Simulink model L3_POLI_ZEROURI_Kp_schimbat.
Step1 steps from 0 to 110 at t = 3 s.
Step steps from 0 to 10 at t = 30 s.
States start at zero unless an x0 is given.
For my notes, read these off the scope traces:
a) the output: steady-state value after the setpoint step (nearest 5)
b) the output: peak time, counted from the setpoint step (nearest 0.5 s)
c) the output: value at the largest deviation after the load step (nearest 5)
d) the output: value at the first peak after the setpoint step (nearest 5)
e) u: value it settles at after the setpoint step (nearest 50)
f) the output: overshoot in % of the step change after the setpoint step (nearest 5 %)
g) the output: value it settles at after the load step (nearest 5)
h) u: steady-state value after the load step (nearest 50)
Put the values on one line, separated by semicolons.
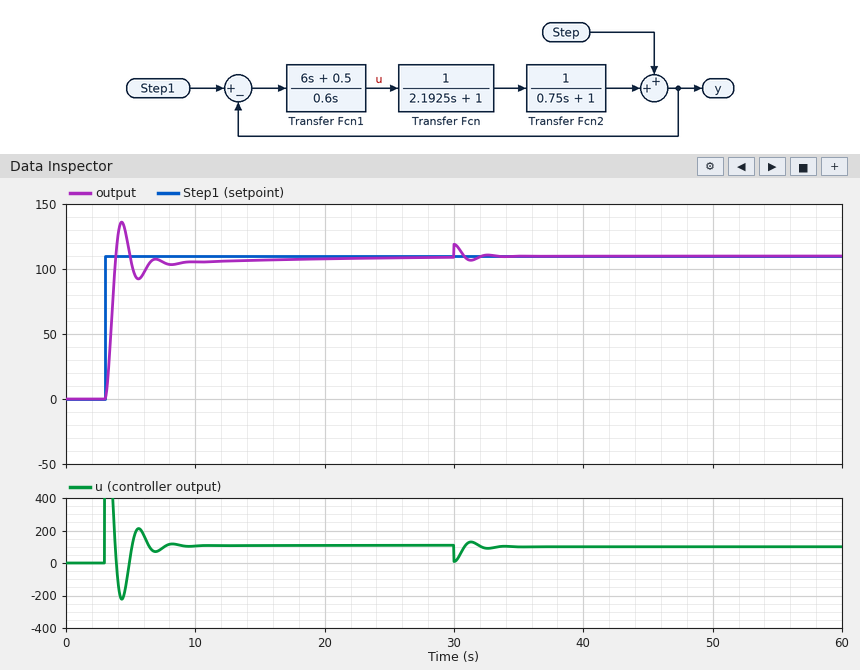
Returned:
110; 1.5 s; 120; 135; 100; 25 %; 110; 100
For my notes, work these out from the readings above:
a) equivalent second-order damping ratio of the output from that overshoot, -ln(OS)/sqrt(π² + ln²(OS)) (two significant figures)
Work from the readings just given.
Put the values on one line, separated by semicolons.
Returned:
0.40
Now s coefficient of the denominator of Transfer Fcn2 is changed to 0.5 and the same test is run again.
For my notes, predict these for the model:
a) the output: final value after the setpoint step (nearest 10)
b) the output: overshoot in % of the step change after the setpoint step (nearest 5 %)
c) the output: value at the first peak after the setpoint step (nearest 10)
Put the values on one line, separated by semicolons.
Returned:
110; 20 %; 130
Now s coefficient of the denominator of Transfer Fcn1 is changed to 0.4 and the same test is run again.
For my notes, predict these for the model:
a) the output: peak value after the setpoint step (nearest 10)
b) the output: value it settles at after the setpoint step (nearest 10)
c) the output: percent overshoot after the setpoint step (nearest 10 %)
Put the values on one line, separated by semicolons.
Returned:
150; 110; 30 %
